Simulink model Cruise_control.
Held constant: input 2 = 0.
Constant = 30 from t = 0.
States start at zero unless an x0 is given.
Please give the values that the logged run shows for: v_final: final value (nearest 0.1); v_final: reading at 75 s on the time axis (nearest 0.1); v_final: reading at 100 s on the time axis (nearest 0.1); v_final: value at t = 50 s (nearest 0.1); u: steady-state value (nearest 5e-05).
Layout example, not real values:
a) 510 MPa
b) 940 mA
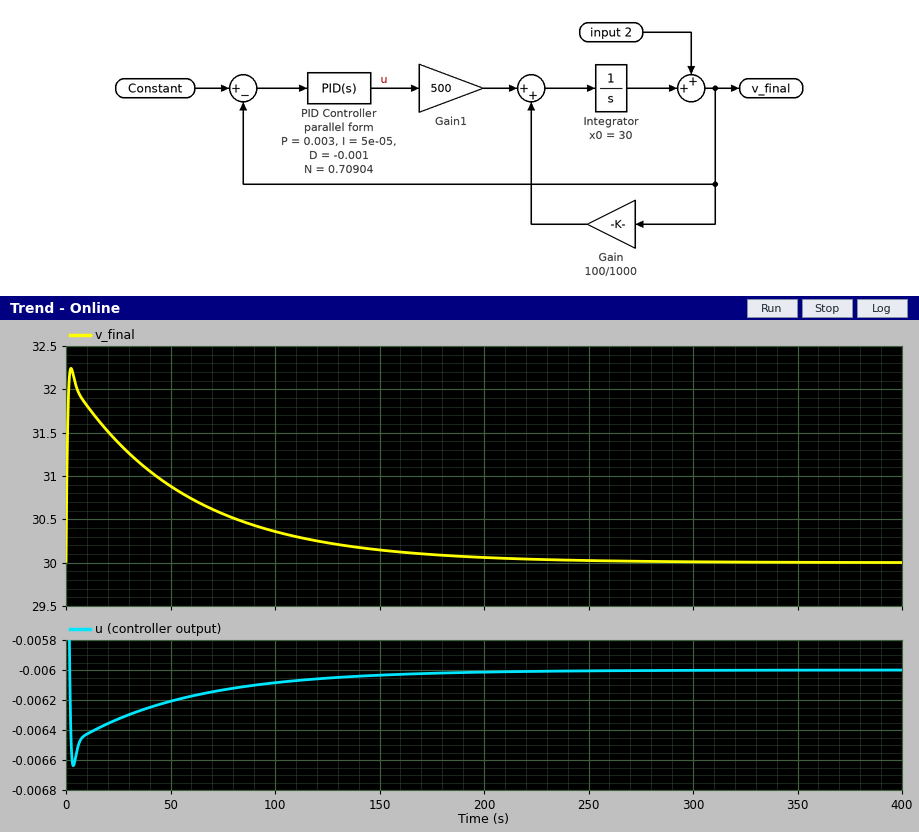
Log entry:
a) 30.0
b) 30.6
c) 30.4
d) 30.9
e) -0.00600
